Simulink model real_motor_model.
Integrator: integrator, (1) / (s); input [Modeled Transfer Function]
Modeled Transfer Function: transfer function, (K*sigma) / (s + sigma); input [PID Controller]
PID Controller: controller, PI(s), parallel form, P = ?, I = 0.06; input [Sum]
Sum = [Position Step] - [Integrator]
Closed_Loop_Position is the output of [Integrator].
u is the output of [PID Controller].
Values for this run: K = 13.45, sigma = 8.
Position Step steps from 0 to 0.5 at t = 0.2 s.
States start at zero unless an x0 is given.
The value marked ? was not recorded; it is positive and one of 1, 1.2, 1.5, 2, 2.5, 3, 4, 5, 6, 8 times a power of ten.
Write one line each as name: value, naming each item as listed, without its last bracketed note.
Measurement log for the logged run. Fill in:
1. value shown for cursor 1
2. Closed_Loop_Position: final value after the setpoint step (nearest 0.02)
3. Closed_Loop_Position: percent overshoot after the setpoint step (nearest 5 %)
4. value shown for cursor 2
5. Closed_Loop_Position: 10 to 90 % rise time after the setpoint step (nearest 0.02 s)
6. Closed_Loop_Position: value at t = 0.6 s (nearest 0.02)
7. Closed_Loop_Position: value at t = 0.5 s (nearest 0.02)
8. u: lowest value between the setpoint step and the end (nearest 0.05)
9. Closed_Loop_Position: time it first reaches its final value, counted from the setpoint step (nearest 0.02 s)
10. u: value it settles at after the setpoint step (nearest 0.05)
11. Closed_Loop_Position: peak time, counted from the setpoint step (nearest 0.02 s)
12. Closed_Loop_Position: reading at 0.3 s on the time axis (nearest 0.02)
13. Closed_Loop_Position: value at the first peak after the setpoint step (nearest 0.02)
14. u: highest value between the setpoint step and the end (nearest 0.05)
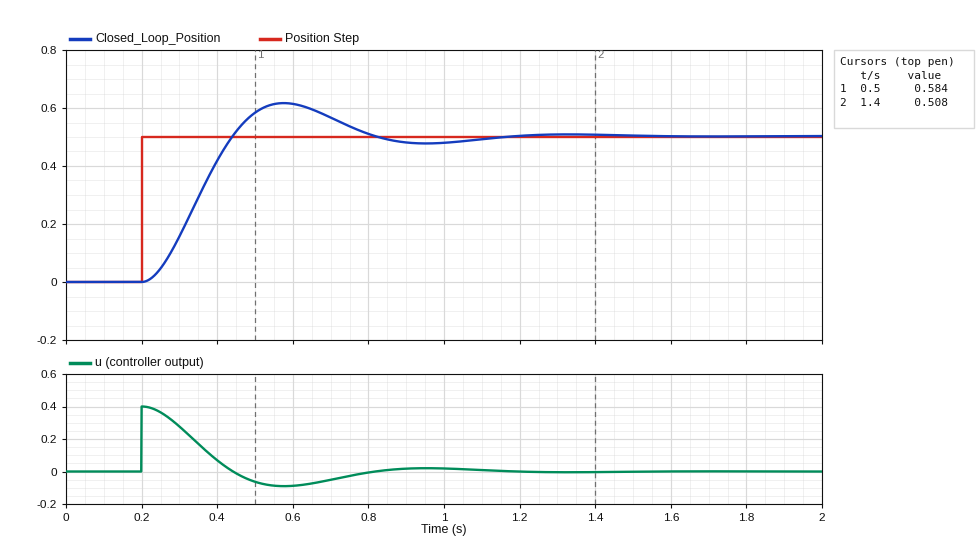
value shown for cursor 1: 0.584
Closed_Loop_Position: final value after the setpoint step: 0.50
Closed_Loop_Position: percent overshoot after the setpoint step: 25 %
value shown for cursor 2: 0.508
Closed_Loop_Position: 10 to 90 % rise time after the setpoint step: 0.16 s
Closed_Loop_Position: value at t = 0.6 s: 0.62
Closed_Loop_Position: value at t = 0.5 s: 0.58
u: lowest value between the setpoint step and the end: -0.10
Closed_Loop_Position: time it first reaches its final value, counted from the setpoint step: 0.24 s
u: value it settles at after the setpoint step: 0.00
Closed_Loop_Position: peak time, counted from the setpoint step: 0.38 s
Closed_Loop_Position: reading at 0.3 s on the time axis: 0.16
Closed_Loop_Position: value at the first peak after the setpoint step: 0.62
u: highest value between the setpoint step and the end: 0.40
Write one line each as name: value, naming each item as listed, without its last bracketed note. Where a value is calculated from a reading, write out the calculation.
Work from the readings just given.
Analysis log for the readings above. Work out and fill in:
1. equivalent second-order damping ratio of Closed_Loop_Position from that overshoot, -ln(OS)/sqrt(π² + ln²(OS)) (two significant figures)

equivalent second-order damping ratio of Closed_Loop_Position from that overshoot, -ln(OS)/sqrt(π² + ln²(OS)): ln(0.25) = -1.386; 1.386 / sqrt(9.870 + 1.922) = 0.40
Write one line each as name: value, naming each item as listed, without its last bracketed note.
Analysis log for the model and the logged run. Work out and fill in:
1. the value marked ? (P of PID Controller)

the value marked ?: 0.8
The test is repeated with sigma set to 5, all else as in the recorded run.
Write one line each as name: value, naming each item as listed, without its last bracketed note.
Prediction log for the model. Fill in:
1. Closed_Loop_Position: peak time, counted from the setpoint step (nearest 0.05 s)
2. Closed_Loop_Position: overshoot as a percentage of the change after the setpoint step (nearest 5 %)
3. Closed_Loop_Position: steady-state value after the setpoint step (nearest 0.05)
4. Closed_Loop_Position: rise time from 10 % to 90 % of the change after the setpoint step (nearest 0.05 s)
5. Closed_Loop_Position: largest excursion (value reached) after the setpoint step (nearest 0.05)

Closed_Loop_Position: peak time, counted from the setpoint step: 0.45 s
Closed_Loop_Position: overshoot as a percentage of the change after the setpoint step: 35 %
Closed_Loop_Position: steady-state value after the setpoint step: 0.50
Closed_Loop_Position: rise time from 10 % to 90 % of the change after the setpoint step: 0.20 s
Closed_Loop_Position: largest excursion (value reached) after the setpoint step: 0.65
